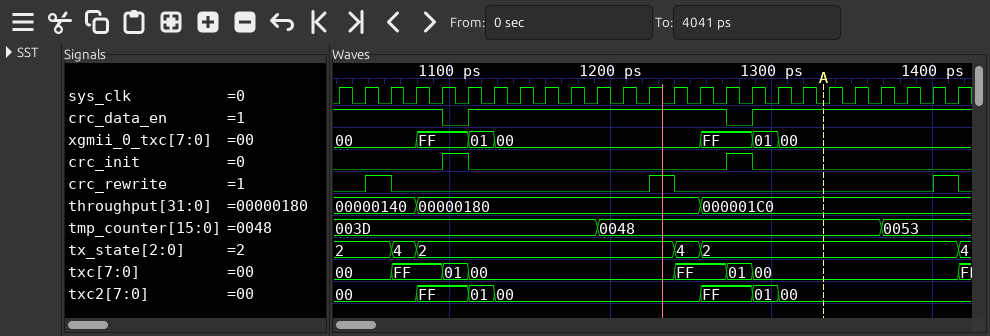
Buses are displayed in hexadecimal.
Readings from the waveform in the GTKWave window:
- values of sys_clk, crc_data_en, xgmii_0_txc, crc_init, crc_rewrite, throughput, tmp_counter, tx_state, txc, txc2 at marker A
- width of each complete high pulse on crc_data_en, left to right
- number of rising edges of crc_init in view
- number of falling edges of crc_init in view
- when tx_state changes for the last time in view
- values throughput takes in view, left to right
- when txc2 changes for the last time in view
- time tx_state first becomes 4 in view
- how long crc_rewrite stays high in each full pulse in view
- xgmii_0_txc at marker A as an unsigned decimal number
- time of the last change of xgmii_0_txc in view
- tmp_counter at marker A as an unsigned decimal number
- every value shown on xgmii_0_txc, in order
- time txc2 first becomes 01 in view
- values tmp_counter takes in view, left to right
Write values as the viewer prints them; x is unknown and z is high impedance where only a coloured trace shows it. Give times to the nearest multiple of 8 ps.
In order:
sys_clk=0, crc_data_en=1, xgmii_0_txc=00, crc_init=0, crc_rewrite=0, throughput=000001C0, tmp_counter=0048, tx_state=2, txc=00, txc2=00
160 ps
2
2
1416 ps
00000140, 00000180, 000001C0
1304 ps
1064 ps
16 ps, 16 ps, 16 ps
0
1304 ps
72
00, FF, 01, 00, FF, 01, 00
1112 ps
003D, 0048, 0053
